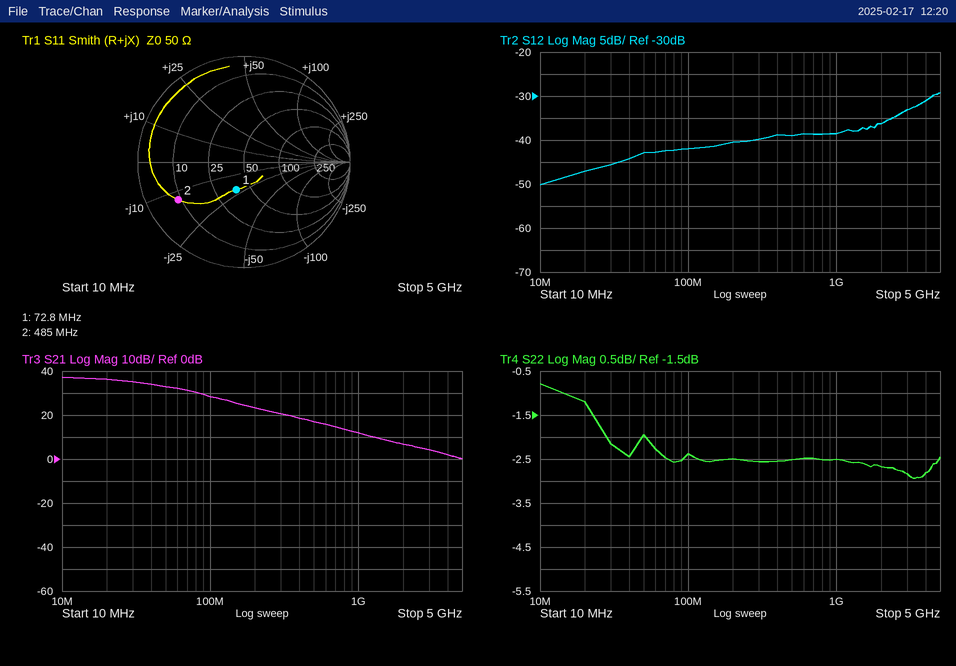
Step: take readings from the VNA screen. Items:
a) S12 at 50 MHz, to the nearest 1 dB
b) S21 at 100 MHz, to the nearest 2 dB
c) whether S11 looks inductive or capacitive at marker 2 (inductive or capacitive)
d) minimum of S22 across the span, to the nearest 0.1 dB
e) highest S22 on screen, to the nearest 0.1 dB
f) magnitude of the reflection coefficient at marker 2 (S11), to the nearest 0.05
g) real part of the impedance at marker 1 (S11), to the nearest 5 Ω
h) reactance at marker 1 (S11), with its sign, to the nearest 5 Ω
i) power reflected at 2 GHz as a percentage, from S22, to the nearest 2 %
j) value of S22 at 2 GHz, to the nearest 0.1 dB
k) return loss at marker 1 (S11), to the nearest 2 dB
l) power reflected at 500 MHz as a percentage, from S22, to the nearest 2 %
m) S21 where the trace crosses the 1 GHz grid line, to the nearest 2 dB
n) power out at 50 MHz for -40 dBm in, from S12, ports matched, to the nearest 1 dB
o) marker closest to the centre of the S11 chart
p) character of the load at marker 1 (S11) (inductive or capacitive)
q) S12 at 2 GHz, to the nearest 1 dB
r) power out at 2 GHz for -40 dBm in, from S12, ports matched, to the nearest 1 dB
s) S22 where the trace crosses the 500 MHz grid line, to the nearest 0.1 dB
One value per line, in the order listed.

-43 dB
28 dB
capacitive
-2.9 dB
-0.8 dB
0.70
40 Ω
-20 Ω
54 %
-2.7 dB
12 dB
56 %
12 dB
-83 dBm
marker 1
capacitive
-36 dB
-76 dBm
-2.5 dB
